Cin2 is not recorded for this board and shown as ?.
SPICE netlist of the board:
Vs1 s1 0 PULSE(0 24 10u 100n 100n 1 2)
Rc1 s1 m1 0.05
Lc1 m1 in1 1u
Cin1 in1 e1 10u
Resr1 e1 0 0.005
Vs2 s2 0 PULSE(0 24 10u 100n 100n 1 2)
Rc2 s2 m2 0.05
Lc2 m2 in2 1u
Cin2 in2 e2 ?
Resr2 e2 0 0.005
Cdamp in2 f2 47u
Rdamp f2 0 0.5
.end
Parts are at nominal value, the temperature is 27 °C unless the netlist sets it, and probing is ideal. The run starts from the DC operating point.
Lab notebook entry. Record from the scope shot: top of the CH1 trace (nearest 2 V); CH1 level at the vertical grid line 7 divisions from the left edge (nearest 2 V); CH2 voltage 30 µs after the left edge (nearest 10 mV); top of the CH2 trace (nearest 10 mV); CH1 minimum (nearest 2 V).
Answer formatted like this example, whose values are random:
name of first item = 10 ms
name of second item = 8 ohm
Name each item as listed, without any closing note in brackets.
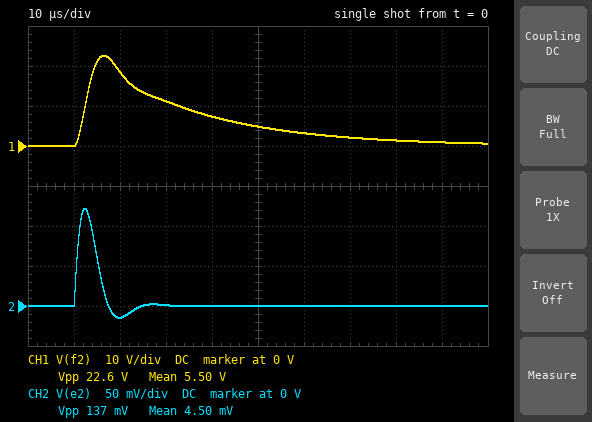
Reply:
top of the CH1 trace = 22 V
CH1 level at the vertical grid line 7 divisions from the left edge = 2 V
CH2 voltage 30 µs after the left edge = 0 V
top of the CH2 trace = 120 mV
CH1 minimum = 0 V
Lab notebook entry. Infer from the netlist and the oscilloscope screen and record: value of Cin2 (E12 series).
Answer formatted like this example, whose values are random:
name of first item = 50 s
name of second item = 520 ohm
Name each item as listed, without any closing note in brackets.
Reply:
value of Cin2 = 3.9 µF
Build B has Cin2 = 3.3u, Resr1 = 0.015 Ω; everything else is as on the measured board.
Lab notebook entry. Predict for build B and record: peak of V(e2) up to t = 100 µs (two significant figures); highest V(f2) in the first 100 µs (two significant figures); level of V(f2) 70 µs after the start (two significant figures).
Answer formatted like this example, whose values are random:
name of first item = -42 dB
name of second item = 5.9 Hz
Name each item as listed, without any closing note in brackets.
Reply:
peak of V(e2) up to t = 100 µs = 110 mV
highest V(f2) in the first 100 µs = 22 V
level of V(f2) 70 µs after the start = 2.1 V
